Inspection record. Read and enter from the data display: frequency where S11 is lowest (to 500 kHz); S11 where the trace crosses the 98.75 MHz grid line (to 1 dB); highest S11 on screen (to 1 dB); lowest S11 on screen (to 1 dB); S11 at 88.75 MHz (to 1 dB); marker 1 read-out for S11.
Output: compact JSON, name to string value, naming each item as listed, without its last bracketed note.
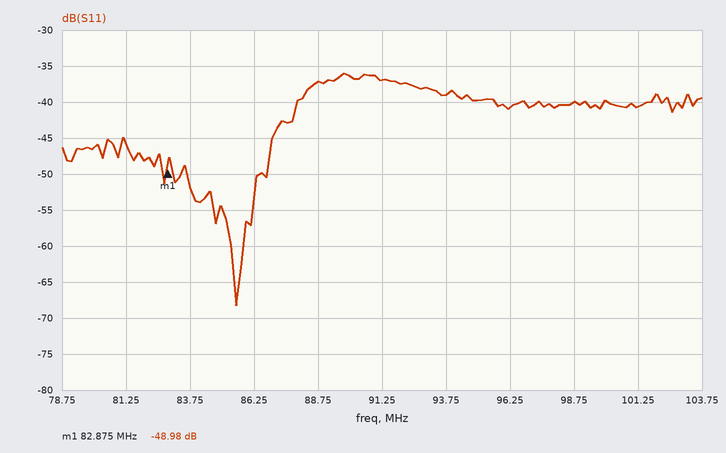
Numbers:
{"frequency where S11 is lowest": "85.5 MHz", "S11 where the trace crosses the 98.75 MHz grid line": "-40 dB", "highest S11 on screen": "-36 dB", "lowest S11 on screen": "-68 dB", "S11 at 88.75 MHz": "-37 dB", "marker 1 read-out for S11": "-48.98 dB"}
